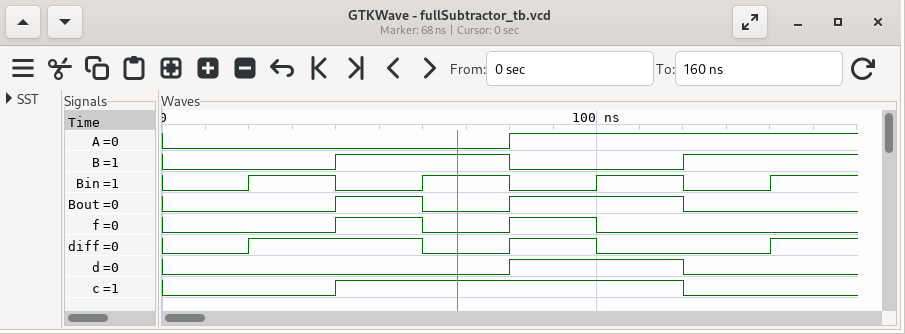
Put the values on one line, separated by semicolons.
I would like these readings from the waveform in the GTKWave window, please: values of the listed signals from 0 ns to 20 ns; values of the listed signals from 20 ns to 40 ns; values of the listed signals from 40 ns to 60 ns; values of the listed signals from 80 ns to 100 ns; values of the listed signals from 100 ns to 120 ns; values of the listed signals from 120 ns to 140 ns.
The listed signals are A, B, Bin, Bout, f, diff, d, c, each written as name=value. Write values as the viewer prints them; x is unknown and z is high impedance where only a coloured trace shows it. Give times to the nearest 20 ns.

A=0, B=0, Bin=0, Bout=0, f=0, diff=0, d=0, c=0; A=0, B=0, Bin=1, Bout=0, f=0, diff=1, d=0, c=0; A=0, B=1, Bin=0, Bout=1, f=1, diff=1, d=0, c=1; A=1, B=0, Bin=0, Bout=1, f=1, diff=1, d=1, c=1; A=1, B=0, Bin=1, Bout=1, f=0, diff=0, d=1, c=1; A=1, B=1, Bin=0, Bout=0, f=0, diff=0, d=0, c=0
